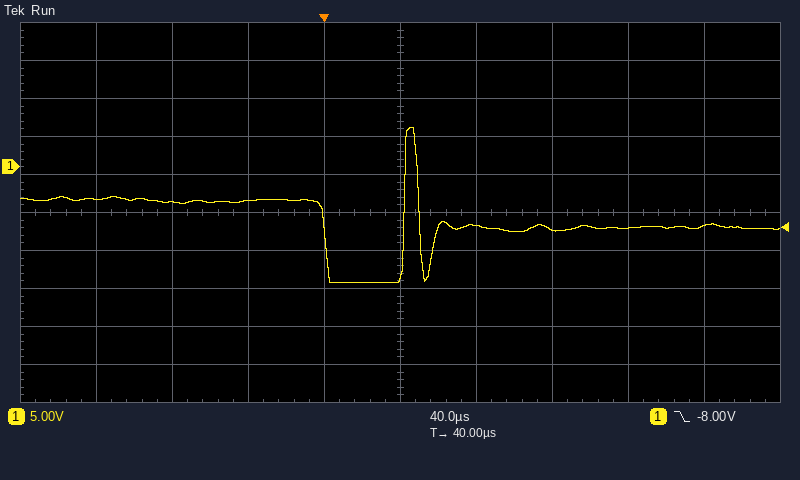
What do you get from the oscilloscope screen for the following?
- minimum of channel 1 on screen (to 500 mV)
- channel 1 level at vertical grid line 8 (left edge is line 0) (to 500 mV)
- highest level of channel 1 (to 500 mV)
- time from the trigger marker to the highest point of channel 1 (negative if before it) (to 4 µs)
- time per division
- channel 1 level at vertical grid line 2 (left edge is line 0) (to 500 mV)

-15.0 V
-8.0 V
5.0 V
+44 µs
40 µs
-4.5 V
